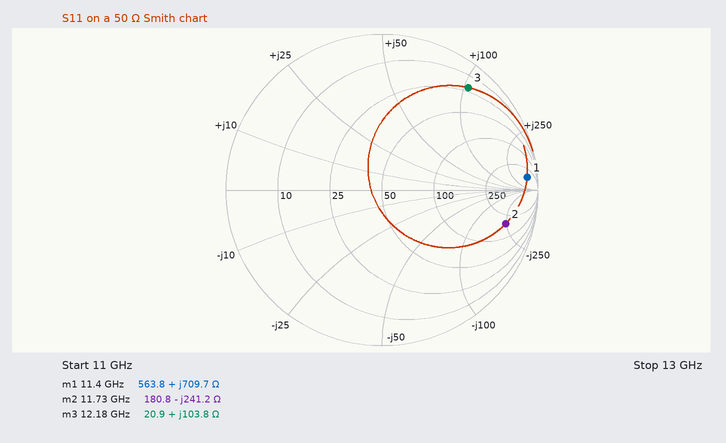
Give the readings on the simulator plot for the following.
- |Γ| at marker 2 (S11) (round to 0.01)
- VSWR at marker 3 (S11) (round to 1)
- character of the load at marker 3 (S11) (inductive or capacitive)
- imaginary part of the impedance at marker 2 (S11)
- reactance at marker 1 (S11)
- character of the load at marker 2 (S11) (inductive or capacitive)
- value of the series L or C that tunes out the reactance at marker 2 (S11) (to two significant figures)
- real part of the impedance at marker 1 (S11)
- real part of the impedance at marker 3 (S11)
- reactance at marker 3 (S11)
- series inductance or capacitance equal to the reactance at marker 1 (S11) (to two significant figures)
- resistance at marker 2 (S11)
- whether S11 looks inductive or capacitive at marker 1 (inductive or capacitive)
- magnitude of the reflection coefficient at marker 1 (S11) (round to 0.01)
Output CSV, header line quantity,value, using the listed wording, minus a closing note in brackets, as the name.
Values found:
quantity,value
|Γ| at marker 2 (S11),0.82
VSWR at marker 3 (S11),13
character of the load at marker 3 (S11),inductive
imaginary part of the impedance at marker 2,-241.2 Ω
reactance at marker 1,+709.7 Ω
character of the load at marker 2 (S11),capacitive
value of the series L or C that tunes out the reactance at marker 2 (S11),3.3 nH
real part of the impedance at marker 1,563.8 Ω
real part of the impedance at marker 3,20.9 Ω
reactance at marker 3,+103.8 Ω
series inductance or capacitance equal to the reactance at marker 1 (S11),9.9 nH
resistance at marker 2,180.8 Ω
whether S11 looks inductive or capacitive at marker 1,inductive
magnitude of the reflection coefficient at marker 1 (S11),0.93
